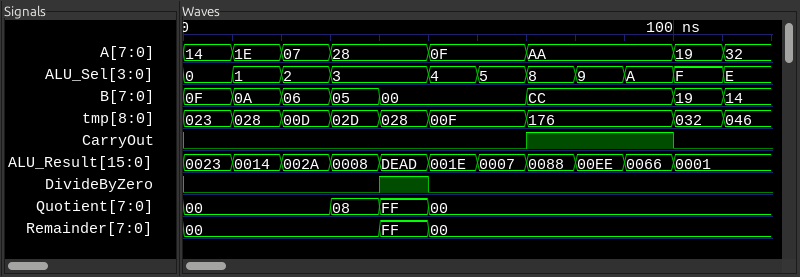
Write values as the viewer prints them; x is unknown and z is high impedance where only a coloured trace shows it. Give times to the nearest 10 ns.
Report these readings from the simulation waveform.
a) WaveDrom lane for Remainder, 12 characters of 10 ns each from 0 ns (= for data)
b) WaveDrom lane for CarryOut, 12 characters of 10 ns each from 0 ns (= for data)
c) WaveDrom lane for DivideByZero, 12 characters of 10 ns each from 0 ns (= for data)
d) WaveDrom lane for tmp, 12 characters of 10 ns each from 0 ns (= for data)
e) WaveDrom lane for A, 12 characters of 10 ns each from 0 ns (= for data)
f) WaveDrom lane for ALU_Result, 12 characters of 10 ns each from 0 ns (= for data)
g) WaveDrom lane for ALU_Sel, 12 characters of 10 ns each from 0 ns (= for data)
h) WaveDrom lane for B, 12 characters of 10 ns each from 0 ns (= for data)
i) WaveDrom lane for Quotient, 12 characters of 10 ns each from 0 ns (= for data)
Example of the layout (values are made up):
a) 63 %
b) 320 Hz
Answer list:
a) {name: 'Remainder', wave: '=...==......', data: '00 FF 00'}
b) {name: 'CarryOut', wave: '0......1..0.'}
c) {name: 'DivideByZero', wave: '0...10......'}
d) {name: 'tmp', wave: '======.=..==', data: '023 028 00D 02D 028 00F 176 032 046'}
e) {name: 'A', wave: '====.=.=..==', data: '14 1E 07 28 0F AA 19 32'}
f) {name: 'ALU_Result', wave: '===========.', data: '0023 0014 002A 0008 DEAD 001E 0007 0088 00EE 0066 0001'}
g) {name: 'ALU_Sel', wave: '====.=======', data: '0 1 2 3 4 5 8 9 A F E'}
h) {name: 'B', wave: '=====..=..==', data: '0F 0A 06 05 00 CC 19 14'}
i) {name: 'Quotient', wave: '=..===......', data: '00 08 FF 00'}
